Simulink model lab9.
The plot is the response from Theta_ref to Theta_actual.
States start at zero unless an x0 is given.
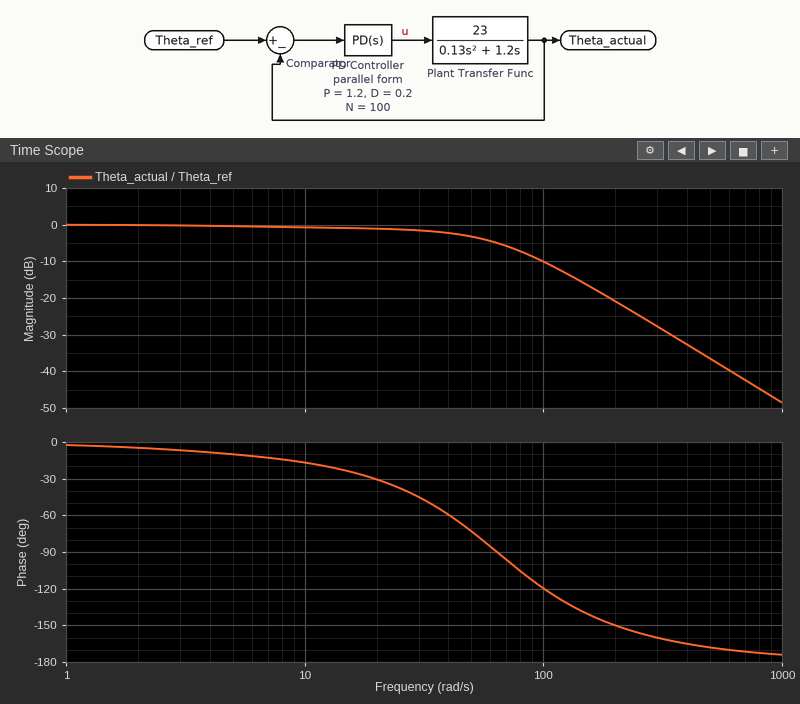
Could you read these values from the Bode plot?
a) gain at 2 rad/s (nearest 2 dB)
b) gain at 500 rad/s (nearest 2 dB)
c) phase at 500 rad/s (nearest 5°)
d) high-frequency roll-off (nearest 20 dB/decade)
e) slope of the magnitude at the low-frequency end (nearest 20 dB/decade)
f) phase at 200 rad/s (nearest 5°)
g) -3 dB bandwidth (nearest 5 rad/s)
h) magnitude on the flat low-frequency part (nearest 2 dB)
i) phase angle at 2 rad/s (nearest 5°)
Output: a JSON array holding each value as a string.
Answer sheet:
["0 dB", "-36 dB", "-170°", "-40 dB/decade", "0 dB/decade", "-150°", "50 rad/s", "0 dB", "-5°"]
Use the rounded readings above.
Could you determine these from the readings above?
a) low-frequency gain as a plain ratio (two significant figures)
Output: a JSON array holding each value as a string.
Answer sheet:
["1.0"]
